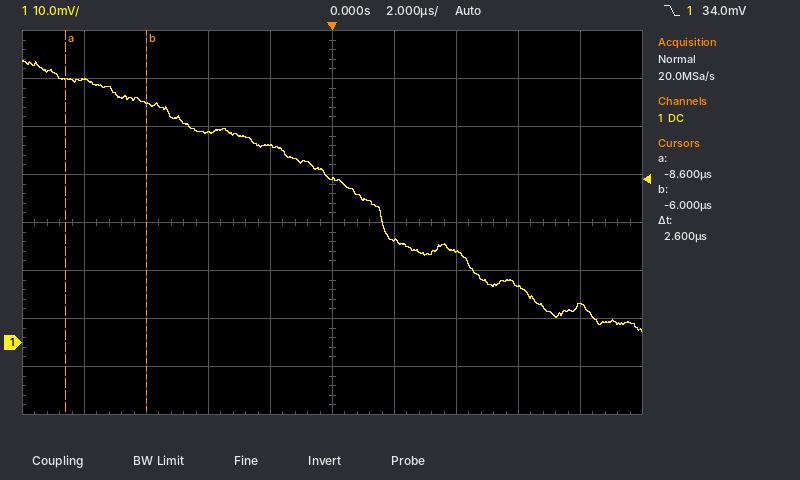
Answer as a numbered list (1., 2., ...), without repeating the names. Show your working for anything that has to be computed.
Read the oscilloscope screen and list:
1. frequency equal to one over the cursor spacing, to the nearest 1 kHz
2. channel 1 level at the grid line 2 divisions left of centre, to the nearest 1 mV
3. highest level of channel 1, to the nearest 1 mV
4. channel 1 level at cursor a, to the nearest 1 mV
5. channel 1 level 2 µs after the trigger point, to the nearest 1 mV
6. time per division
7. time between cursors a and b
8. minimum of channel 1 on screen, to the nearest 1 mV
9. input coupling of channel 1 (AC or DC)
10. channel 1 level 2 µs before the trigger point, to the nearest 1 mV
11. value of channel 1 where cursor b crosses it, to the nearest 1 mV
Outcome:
1. 1 / 2.6 µs ≈ 385 kHz
2. 44 mV
3. 59 mV
4. 55 mV
5. 21 mV
6. 2 µs
7. 2.6 µs
8. 2 mV
9. DC
10. 41 mV
11. 50 mV
